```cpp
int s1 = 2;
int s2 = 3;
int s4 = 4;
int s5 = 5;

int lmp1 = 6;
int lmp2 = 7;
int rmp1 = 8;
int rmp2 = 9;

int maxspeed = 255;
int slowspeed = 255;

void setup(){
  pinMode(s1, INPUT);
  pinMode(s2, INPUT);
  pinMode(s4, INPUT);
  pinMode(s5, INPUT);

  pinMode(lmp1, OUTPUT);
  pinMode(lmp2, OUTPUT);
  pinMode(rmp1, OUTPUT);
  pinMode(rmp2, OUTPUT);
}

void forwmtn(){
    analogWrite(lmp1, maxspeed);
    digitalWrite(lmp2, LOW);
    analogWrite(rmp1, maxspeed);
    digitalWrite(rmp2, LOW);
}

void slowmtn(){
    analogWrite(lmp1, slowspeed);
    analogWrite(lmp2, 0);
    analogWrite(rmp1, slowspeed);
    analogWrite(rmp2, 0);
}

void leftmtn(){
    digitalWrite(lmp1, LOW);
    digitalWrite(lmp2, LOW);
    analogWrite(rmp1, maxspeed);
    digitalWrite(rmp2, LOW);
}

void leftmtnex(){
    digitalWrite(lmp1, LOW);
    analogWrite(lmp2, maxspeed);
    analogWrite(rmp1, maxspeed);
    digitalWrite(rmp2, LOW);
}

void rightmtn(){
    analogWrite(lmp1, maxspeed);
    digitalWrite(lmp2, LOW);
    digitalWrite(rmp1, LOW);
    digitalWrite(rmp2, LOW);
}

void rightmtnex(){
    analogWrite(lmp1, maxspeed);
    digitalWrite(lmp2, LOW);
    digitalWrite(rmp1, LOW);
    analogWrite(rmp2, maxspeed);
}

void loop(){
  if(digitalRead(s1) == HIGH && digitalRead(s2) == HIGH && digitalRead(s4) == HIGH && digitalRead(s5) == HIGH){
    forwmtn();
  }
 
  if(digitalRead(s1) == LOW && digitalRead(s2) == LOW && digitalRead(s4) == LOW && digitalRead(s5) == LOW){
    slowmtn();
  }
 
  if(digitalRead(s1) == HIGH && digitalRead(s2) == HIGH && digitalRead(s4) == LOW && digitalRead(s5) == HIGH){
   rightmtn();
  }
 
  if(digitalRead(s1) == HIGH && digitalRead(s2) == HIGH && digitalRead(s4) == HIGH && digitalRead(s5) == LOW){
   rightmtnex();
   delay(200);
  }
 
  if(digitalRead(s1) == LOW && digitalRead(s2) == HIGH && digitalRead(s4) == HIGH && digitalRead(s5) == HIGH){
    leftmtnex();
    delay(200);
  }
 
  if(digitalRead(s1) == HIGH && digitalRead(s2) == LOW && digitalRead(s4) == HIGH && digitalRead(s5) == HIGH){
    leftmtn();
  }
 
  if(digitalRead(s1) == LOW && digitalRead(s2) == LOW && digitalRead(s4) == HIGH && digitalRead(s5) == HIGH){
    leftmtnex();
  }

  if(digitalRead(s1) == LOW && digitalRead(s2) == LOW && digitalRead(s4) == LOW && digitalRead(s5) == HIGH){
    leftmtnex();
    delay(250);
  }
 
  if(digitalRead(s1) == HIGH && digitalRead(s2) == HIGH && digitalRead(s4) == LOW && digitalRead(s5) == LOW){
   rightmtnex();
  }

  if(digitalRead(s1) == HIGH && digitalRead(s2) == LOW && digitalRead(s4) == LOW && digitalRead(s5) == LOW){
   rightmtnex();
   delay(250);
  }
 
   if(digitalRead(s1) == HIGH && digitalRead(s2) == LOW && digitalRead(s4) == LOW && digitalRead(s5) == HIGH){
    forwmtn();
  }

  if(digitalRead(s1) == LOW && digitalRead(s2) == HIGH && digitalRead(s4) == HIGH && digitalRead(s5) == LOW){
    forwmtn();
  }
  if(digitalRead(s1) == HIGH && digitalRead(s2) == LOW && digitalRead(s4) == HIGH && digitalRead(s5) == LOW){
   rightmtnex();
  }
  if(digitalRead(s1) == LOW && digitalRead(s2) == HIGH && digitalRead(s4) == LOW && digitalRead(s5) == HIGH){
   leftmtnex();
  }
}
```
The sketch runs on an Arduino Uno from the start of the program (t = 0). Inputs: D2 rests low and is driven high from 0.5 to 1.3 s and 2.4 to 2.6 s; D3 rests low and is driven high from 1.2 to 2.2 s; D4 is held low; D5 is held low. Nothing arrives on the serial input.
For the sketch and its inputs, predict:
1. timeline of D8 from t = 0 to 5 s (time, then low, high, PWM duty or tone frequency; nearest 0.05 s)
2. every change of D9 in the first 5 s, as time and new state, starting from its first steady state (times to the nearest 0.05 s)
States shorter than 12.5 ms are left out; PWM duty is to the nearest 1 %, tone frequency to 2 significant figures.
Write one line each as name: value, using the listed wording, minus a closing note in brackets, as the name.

timeline of D8 from t = 0 to 5 s: 0 s high; 0.5 s low; 2.2 s high; 2.4 s low; 2.65 s high
every change of D9 in the first 5 s, as time and new state, starting from its first steady state: 0 s low; 0.5 s high; 2.2 s low; 2.4 s high; 2.65 s low
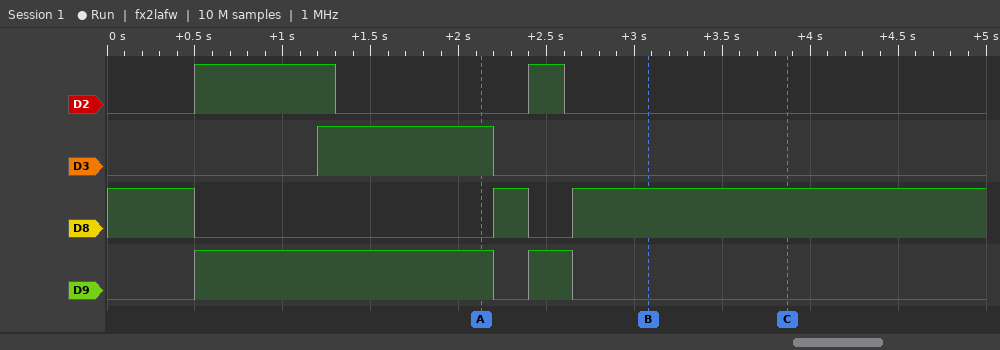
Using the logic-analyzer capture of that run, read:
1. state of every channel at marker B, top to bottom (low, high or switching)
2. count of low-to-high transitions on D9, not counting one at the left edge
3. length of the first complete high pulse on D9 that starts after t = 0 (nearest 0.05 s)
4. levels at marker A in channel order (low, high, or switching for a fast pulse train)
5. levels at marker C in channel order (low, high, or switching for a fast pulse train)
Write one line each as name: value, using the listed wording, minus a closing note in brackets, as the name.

state of every channel at marker B, top to bottom: D2 low, D3 low, D8 high, D9 low
count of low-to-high transitions on D9, not counting one at the left edge: 2
length of the first complete high pulse on D9 that starts after t = 0: 1.70 s
levels at marker A in channel order: D2 low, D3 high, D8 low, D9 high
levels at marker C in channel order: D2 low, D3 low, D8 high, D9 low
